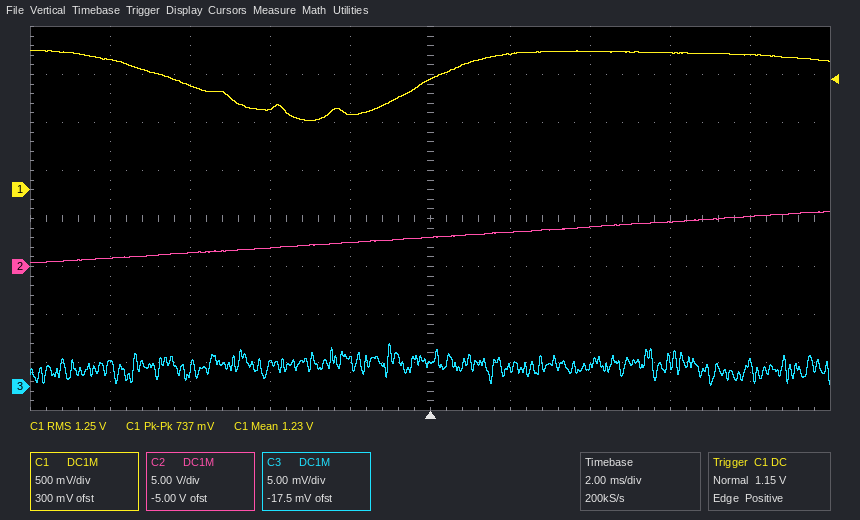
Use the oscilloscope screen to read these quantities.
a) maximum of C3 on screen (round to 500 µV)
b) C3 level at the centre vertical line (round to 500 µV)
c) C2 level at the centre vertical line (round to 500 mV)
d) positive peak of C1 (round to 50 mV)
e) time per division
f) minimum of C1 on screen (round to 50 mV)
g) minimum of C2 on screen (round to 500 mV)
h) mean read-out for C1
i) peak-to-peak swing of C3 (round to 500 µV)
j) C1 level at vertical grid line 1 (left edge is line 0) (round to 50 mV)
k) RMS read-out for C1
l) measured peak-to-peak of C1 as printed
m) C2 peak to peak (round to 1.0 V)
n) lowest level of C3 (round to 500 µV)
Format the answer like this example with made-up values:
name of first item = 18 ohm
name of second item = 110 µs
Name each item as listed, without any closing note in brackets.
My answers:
maximum of C3 on screen = 4.5 mV
C3 level at the centre vertical line = 2.5 mV
C2 level at the centre vertical line = 3.0 V
positive peak of C1 = 1.45 V
time per division = 2 ms
minimum of C1 on screen = 700 mV
minimum of C2 on screen = 500 mV
mean read-out for C1 = 1.23 V
peak-to-peak swing of C3 = 4.5 mV
C1 level at vertical grid line 1 (left edge is line 0) = 1.35 V
RMS read-out for C1 = 1.25 V
measured peak-to-peak of C1 as printed = 737 mV
C2 peak to peak = 5.0 V
lowest level of C3 = 0.0 mV
